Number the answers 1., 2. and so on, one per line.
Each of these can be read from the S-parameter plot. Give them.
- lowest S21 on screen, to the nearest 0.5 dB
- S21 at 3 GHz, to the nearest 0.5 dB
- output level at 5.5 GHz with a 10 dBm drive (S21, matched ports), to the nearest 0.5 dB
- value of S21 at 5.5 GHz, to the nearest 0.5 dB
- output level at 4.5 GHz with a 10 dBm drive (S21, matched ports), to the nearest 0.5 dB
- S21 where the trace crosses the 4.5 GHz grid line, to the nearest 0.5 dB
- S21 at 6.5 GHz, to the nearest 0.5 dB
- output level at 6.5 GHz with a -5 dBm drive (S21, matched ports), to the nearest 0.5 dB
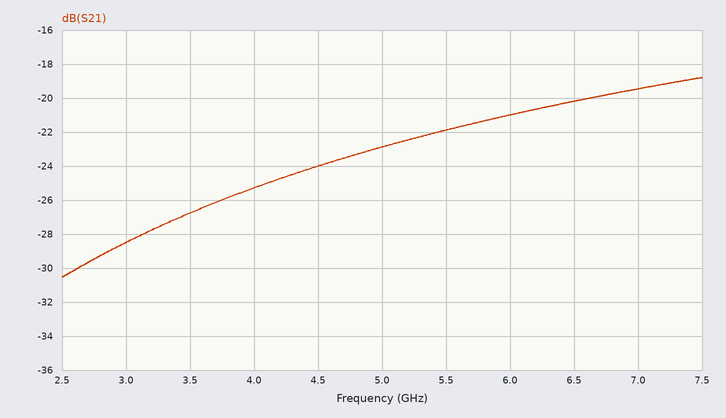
1. -30.5 dB
2. -28.5 dB
3. -12.0 dBm
4. -22.0 dB
5. -14.0 dBm
6. -24.0 dB
7. -20.0 dB
8. -25.0 dBm
